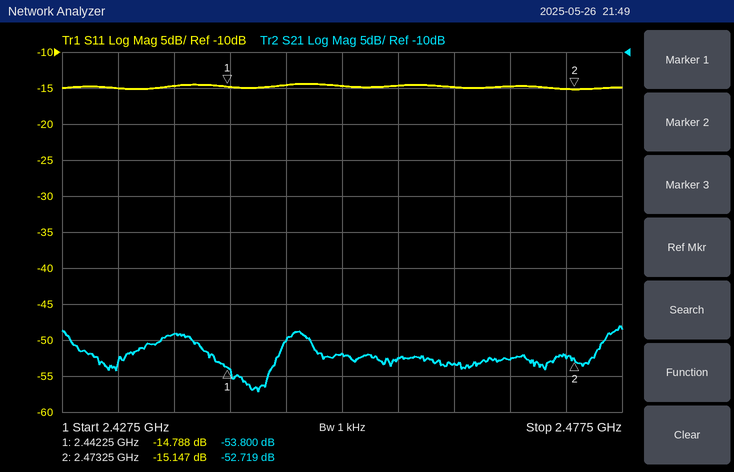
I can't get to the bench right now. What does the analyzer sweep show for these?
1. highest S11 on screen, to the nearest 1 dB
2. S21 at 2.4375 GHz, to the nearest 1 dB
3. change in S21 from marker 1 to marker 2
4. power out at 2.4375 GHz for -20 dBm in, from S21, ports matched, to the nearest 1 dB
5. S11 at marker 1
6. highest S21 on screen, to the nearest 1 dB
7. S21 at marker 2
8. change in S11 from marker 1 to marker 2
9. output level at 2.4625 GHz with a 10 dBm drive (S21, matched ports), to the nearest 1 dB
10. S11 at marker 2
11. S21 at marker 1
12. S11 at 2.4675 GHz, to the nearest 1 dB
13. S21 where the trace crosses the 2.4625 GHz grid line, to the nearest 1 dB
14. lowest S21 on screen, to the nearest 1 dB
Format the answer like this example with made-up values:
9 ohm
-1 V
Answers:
-14 dB
-49 dB
1.081 dB
-69 dBm
-14.788 dB
-48 dB
-52.719 dB
-0.359 dB
-43 dBm
-15.147 dB
-53.800 dB
-15 dB
-53 dB
-57 dB
